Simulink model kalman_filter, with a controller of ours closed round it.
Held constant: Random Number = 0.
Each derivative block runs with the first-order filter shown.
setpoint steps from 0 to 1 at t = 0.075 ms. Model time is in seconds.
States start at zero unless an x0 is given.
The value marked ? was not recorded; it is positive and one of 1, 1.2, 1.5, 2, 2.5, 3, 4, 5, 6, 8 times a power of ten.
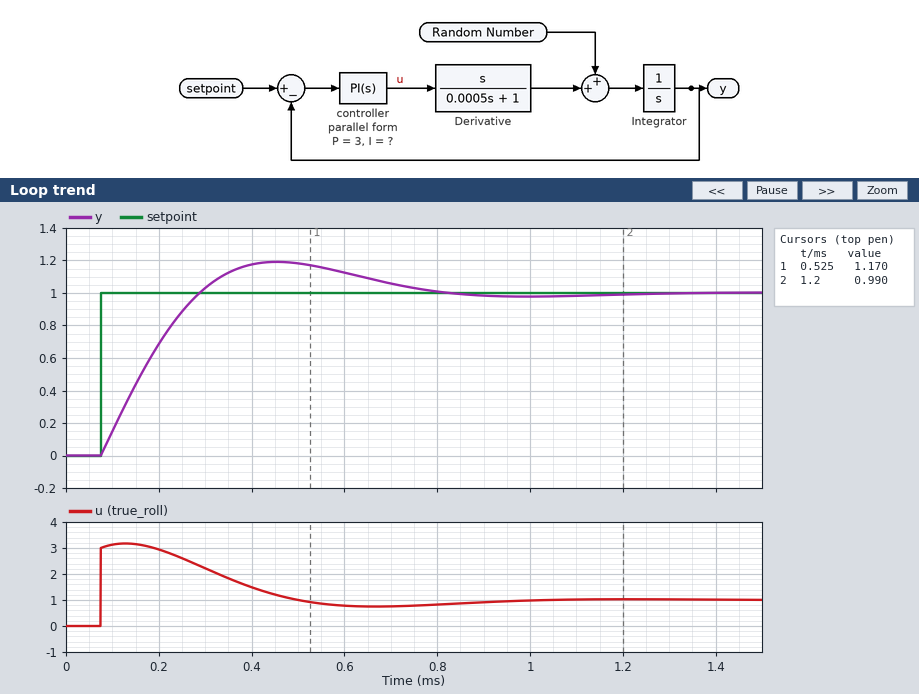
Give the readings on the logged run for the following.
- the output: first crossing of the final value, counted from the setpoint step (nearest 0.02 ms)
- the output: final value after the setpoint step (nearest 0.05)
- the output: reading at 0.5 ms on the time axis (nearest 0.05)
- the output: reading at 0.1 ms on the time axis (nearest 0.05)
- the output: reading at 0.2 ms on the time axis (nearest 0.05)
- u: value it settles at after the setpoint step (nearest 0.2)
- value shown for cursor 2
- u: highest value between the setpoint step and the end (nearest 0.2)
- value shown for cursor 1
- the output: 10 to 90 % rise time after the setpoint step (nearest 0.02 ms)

0.22 ms
1.00
1.20
0.15
0.70
1.0
0.990
3.2
1.170
0.16 ms
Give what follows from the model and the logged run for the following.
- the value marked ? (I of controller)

25000
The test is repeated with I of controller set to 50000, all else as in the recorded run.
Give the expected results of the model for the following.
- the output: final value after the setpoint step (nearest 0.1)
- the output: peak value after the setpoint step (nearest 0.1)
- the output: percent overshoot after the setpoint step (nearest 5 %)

1.0
1.3
30 %
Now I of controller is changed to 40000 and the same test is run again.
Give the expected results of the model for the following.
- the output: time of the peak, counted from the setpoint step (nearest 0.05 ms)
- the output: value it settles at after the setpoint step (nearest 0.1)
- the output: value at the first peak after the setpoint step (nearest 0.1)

0.30 ms
1.0
1.3
